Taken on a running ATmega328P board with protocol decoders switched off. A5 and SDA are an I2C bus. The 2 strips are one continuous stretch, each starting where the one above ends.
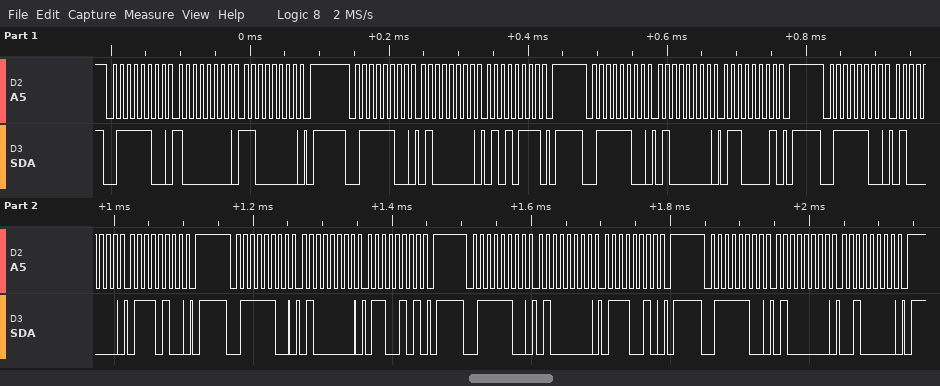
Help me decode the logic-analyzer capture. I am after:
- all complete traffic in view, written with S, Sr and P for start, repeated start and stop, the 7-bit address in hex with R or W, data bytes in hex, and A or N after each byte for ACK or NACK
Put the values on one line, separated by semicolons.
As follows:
S 3EW A 80 A C0 A P S 3EW A 40 A 57 A P S 3EW A 40 A 61 A P S 3EW A 40 A 74 A P S 3EW A 40 A 65 A P S 3EW A 40 A 72 A P S 3EW A 40 A 20 A P
